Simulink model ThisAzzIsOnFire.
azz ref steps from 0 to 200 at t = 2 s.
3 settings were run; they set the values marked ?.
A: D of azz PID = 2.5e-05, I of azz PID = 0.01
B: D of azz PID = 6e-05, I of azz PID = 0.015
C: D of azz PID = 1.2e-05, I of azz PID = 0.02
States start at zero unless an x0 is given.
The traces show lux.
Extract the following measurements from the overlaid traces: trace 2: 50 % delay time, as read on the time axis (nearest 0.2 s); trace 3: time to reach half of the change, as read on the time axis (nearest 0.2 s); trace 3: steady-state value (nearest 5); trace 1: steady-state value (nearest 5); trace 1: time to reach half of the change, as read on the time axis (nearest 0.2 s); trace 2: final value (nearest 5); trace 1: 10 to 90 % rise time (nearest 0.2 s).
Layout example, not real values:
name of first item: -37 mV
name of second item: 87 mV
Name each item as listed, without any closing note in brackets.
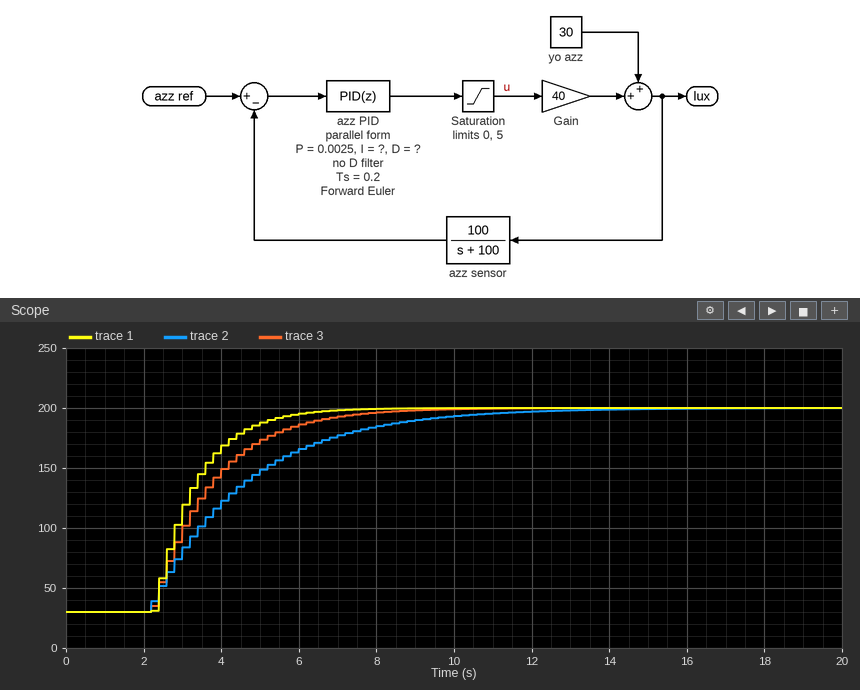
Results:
trace 2: 50 % delay time, as read on the time axis: 3.8 s
trace 3: time to reach half of the change, as read on the time axis: 3.4 s
trace 3: steady-state value: 200
trace 1: steady-state value: 200
trace 1: time to reach half of the change, as read on the time axis: 3.0 s
trace 2: final value: 200
trace 1: 10 to 90 % rise time: 2.4 s
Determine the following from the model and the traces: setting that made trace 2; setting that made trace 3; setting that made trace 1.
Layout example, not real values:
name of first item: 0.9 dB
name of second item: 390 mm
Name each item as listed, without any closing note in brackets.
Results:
setting that made trace 2: A
setting that made trace 3: B
setting that made trace 1: C
